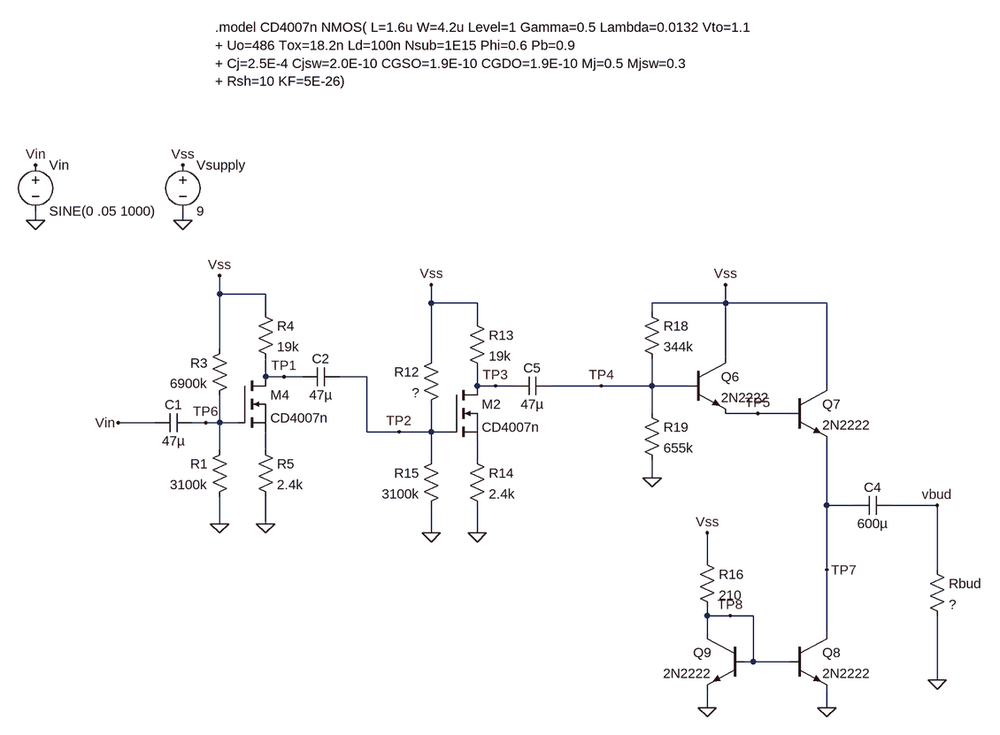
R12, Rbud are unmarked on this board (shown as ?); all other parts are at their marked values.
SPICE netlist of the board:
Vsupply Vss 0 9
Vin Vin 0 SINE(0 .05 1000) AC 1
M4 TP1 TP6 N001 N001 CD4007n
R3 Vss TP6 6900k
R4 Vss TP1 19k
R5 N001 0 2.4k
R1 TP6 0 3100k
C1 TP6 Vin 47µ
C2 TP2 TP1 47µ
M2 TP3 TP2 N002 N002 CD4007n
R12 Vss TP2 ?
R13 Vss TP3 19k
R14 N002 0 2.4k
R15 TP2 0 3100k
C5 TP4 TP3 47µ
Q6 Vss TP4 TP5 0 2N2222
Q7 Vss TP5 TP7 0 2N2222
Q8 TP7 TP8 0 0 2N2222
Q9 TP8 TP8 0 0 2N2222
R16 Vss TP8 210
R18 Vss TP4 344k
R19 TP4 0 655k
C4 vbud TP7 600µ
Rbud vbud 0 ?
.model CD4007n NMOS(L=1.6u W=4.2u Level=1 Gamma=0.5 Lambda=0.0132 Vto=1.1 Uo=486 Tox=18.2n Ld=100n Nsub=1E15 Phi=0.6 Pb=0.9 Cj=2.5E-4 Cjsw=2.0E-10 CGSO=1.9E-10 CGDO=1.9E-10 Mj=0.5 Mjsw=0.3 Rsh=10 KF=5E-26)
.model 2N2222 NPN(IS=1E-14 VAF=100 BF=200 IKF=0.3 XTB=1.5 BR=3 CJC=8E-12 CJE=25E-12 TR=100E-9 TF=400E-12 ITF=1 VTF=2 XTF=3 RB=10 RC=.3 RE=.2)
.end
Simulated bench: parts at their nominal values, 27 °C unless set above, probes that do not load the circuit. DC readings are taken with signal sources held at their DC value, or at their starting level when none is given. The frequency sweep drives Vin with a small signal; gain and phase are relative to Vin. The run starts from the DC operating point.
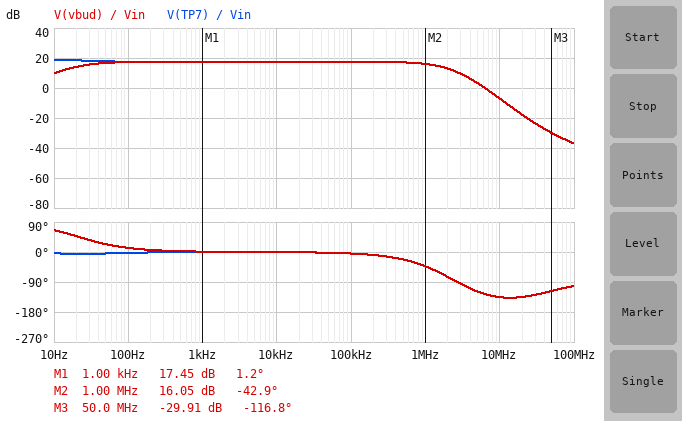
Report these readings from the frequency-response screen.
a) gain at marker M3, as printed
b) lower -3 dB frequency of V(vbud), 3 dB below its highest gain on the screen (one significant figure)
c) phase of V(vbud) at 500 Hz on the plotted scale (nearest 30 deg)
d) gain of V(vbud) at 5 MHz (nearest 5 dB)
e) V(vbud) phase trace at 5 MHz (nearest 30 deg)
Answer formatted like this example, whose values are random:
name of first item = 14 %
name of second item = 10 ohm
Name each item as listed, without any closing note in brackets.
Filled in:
gain at marker M3, as printed = -29.91 dB
lower -3 dB frequency of V(vbud), 3 dB below its highest gain on the screen = 20 Hz
phase of V(vbud) at 500 Hz on the plotted scale = 0 deg
gain of V(vbud) at 5 MHz = 5 dB
V(vbud) phase trace at 5 MHz = -120 deg
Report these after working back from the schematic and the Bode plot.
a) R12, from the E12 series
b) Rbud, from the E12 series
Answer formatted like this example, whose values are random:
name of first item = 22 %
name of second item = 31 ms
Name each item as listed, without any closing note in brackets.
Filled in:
R12, from the E12 series = 10 MΩ
Rbud, from the E12 series = 10 Ω
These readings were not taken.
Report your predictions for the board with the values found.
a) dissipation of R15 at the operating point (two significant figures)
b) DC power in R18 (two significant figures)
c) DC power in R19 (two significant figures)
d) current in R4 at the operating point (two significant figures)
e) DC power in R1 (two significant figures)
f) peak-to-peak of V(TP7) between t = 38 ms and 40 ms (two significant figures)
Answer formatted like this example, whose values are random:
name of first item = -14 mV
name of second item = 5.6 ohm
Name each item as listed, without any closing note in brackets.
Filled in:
dissipation of R15 at the operating point = 1.5 µW
DC power in R18 = 32 µW
DC power in R19 = 49 µW
current in R4 at the operating point = 210 µA
DC power in R1 = 2.5 µW
peak-to-peak of V(TP7) between t = 38 ms and 40 ms = 710 mV
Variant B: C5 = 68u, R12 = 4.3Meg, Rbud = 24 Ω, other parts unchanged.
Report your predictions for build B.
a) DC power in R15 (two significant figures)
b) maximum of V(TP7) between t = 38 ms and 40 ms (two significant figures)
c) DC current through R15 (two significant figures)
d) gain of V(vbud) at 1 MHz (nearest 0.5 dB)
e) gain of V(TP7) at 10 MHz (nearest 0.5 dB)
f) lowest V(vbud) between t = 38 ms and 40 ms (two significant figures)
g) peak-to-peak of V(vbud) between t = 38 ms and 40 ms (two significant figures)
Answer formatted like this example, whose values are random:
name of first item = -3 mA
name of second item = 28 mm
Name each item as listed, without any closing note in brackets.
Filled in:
DC power in R15 = 4.6 µW
maximum of V(TP7) between t = 38 ms and 40 ms = 4.5 V
DC current through R15 = 1.2 µA
gain of V(vbud) at 1 MHz = 9.0 dB
gain of V(TP7) at 10 MHz = -2.5 dB
lowest V(vbud) between t = 38 ms and 40 ms = -130 mV
peak-to-peak of V(vbud) between t = 38 ms and 40 ms = 310 mV
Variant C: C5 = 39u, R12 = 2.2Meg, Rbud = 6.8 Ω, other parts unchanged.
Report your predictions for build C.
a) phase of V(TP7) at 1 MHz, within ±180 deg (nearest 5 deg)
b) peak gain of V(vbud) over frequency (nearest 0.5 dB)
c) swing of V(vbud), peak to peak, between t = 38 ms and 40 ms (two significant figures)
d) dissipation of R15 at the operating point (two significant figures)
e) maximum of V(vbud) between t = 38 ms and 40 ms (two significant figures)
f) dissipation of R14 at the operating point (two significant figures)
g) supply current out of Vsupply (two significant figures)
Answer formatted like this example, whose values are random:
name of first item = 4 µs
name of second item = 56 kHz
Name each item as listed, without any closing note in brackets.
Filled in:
phase of V(TP7) at 1 MHz, within ±180 deg = -15 deg
peak gain of V(vbud) over frequency = -8.0 dB
swing of V(vbud), peak to peak, between t = 38 ms and 40 ms = 39 mV
dissipation of R15 at the operating point = 8.9 µW
maximum of V(vbud) between t = 38 ms and 40 ms = 20 mV
dissipation of R14 at the operating point = 380 µW
supply current out of Vsupply = 80 mA
